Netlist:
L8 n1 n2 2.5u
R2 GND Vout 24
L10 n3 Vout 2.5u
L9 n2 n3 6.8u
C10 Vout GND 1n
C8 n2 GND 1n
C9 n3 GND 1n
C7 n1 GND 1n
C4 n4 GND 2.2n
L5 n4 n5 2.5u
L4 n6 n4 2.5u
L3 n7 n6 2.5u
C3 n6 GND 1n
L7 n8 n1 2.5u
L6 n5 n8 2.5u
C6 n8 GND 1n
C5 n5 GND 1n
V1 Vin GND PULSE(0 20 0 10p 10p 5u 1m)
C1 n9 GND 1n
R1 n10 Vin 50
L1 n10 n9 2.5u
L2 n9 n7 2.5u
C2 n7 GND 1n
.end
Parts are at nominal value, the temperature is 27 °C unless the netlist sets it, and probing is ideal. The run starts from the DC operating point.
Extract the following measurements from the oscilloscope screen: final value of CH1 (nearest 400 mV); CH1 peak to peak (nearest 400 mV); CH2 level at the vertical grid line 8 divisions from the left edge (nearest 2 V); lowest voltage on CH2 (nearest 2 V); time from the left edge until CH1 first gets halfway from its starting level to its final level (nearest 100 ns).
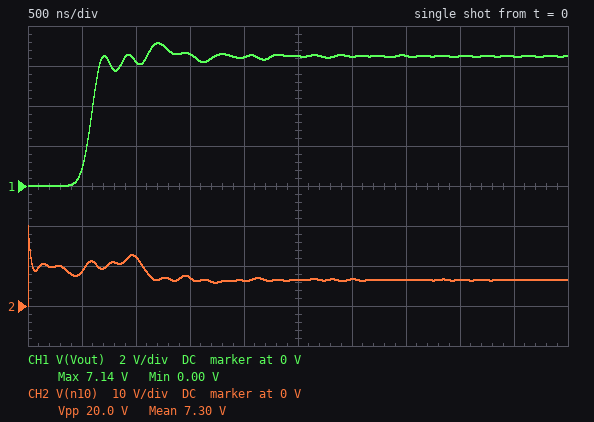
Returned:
6.4 V
7.2 V
6 V
0 V
600 ns
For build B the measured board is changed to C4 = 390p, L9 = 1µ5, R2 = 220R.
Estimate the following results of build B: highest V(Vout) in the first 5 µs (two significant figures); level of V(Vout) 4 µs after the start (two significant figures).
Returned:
19 V
16 V
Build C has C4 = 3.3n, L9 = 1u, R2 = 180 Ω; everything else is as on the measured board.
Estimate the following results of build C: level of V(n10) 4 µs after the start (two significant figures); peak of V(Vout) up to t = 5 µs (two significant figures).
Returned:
16 V
17 V
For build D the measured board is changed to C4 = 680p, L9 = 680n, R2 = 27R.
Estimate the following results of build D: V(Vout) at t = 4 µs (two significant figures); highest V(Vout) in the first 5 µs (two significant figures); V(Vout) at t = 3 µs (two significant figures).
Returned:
7.0 V
8.4 V
7.1 V
